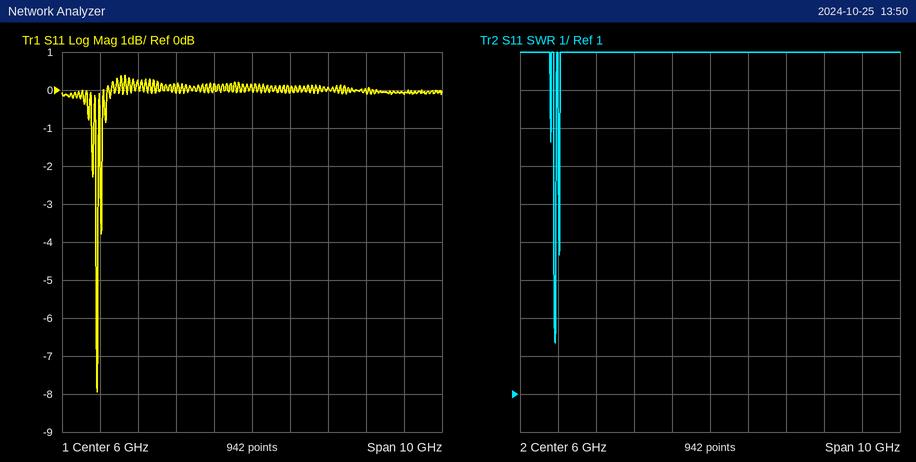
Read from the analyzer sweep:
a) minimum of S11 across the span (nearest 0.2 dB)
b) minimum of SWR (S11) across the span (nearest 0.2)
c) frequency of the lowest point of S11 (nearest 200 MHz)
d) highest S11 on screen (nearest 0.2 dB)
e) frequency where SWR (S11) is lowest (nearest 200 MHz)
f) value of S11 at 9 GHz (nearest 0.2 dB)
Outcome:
-8.0 dB
2.4
2.0 GHz
0.4 dB
2.0 GHz
0.0 dB
